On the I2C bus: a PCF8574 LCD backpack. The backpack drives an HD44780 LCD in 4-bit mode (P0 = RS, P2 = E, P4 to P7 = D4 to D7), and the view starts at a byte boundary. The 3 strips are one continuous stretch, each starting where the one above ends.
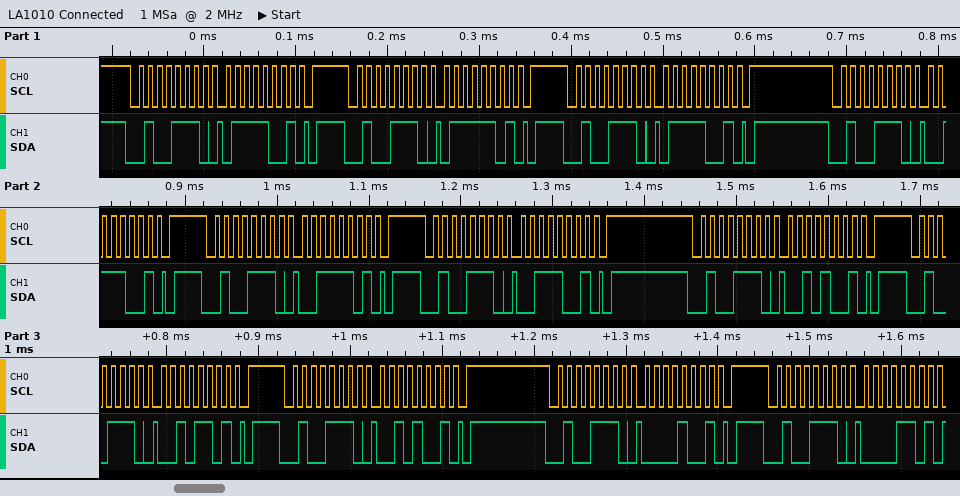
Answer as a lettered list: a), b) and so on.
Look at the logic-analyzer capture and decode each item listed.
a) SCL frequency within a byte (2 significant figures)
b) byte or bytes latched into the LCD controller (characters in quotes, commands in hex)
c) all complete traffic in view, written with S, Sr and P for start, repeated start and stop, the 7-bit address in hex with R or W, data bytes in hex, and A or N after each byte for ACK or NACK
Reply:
a) 100 kHz
b) 's'
c) S 27W A 79 A P S 27W A 7D A P S 27W A 79 A P S 27W A 39 A P S 27W A 3D A P S 27W A 39 A P S 27W A 29 A P S 27W A 2D A P S 27W A 29 A P S 27W A 09 A P S 27W A 0D A
